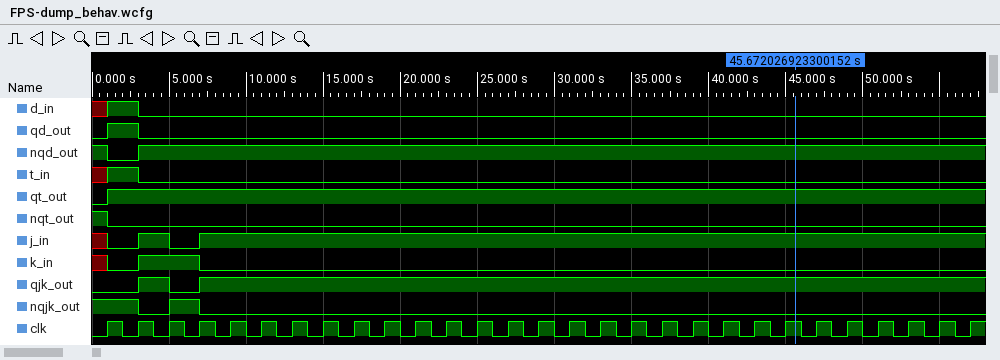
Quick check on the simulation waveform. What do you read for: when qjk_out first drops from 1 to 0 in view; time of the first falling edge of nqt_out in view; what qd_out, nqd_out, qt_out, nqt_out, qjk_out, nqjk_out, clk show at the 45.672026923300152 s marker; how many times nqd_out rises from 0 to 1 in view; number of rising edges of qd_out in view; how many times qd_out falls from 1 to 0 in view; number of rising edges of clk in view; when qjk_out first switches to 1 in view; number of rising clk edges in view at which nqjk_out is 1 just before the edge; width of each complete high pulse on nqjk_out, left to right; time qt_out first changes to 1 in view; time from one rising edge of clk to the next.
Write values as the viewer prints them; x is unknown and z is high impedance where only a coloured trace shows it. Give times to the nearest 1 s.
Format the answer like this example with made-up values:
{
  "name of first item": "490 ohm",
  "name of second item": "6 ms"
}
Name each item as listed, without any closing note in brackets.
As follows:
{
  "when qjk_out first drops from 1 to 0 in view": "5 s",
  "time of the first falling edge of nqt_out in view": "1 s",
  "what qd_out, nqd_out, qt_out, nqt_out, qjk_out, nqjk_out, clk show at the 45.672026923300152 s marker": "qd_out=0, nqd_out=1, qt_out=1, nqt_out=0, qjk_out=1, nqjk_out=0, clk=1",
  "how many times nqd_out rises from 0 to 1 in view": "1",
  "number of rising edges of qd_out in view": "1",
  "how many times qd_out falls from 1 to 0 in view": "1",
  "number of rising edges of clk in view": "29",
  "when qjk_out first switches to 1 in view": "3 s",
  "number of rising clk edges in view at which nqjk_out is 1 just before the edge": "3",
  "width of each complete high pulse on nqjk_out, left to right": "2 s",
  "time qt_out first changes to 1 in view": "1 s",
  "time from one rising edge of clk to the next": "2 s"
}
